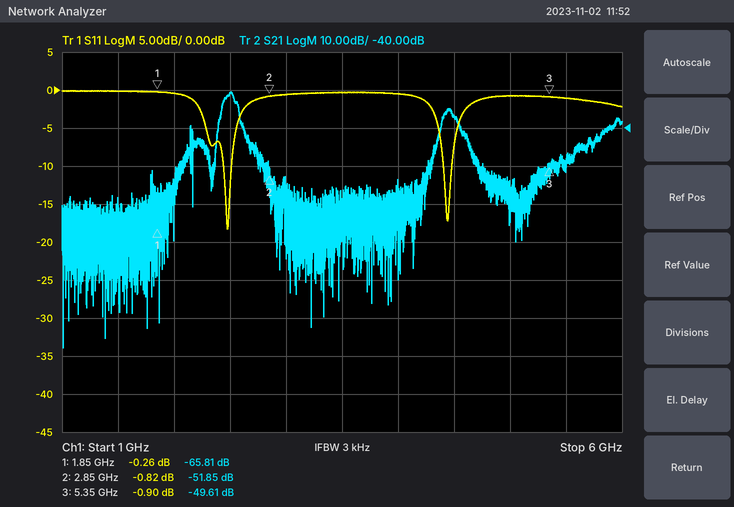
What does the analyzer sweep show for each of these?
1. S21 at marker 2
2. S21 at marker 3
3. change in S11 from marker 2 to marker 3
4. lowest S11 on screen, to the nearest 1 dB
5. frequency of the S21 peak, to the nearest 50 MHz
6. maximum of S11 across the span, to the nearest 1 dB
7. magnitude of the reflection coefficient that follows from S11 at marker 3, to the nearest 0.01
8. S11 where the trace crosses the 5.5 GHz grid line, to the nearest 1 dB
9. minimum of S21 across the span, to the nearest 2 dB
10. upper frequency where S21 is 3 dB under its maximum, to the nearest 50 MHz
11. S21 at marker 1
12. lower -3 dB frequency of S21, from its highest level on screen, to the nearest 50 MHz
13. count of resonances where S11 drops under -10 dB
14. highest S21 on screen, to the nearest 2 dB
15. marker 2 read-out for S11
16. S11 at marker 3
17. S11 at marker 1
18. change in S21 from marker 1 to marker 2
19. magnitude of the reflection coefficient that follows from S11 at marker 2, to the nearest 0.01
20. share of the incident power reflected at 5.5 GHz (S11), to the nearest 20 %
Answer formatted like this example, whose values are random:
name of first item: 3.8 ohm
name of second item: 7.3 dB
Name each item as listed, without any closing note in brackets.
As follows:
S21 at marker 2: -51.85 dB
S21 at marker 3: -49.61 dB
change in S11 from marker 2 to marker 3: -0.08 dB
lowest S11 on screen, to the nearest 1 dB: -18 dB
frequency of the S21 peak, to the nearest 50 MHz: 2.50 GHz
maximum of S11 across the span, to the nearest 1 dB: 0 dB
magnitude of the reflection coefficient that follows from S11 at marker 3, to the nearest 0.01: 0.90
S11 where the trace crosses the 5.5 GHz grid line, to the nearest 1 dB: -1 dB
minimum of S21 across the span, to the nearest 2 dB: -98 dB
upper frequency where S21 is 3 dB under its maximum, to the nearest 50 MHz: 2.55 GHz
S21 at marker 1: -65.81 dB
lower -3 dB frequency of S21, from its highest level on screen, to the nearest 50 MHz: 2.45 GHz
count of resonances where S11 drops under -10 dB: 2
highest S21 on screen, to the nearest 2 dB: -30 dB
marker 2 read-out for S11: -0.82 dB
S11 at marker 3: -0.90 dB
S11 at marker 1: -0.26 dB
change in S21 from marker 1 to marker 2: 13.96 dB
magnitude of the reflection coefficient that follows from S11 at marker 2, to the nearest 0.01: 0.91
share of the incident power reflected at 5.5 GHz (S11), to the nearest 20 %: 80 %
